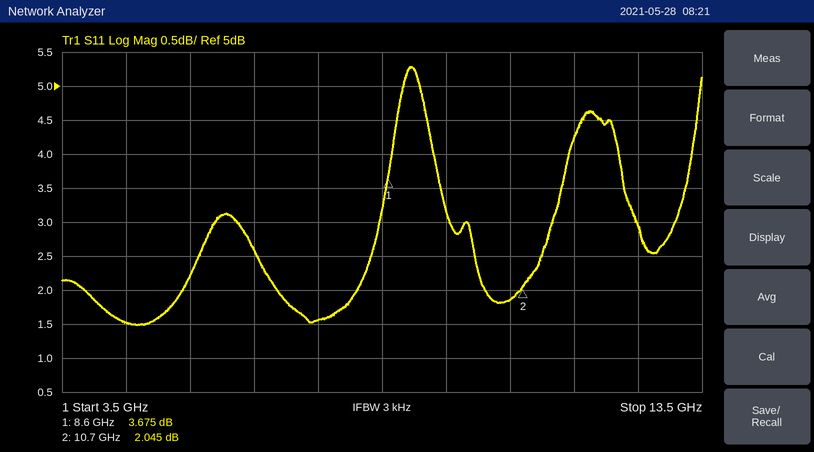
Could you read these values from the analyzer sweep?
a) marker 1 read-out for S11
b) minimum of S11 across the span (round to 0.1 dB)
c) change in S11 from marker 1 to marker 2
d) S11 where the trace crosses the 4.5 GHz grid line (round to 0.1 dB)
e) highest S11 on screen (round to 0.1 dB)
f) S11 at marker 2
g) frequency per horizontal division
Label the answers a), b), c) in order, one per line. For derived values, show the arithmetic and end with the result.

a) 3.675 dB
b) 1.5 dB
c) 2.045 − (3.675) = -1.630 dB
d) 1.5 dB
e) 5.3 dB
f) 2.045 dB
g) 1 GHz
